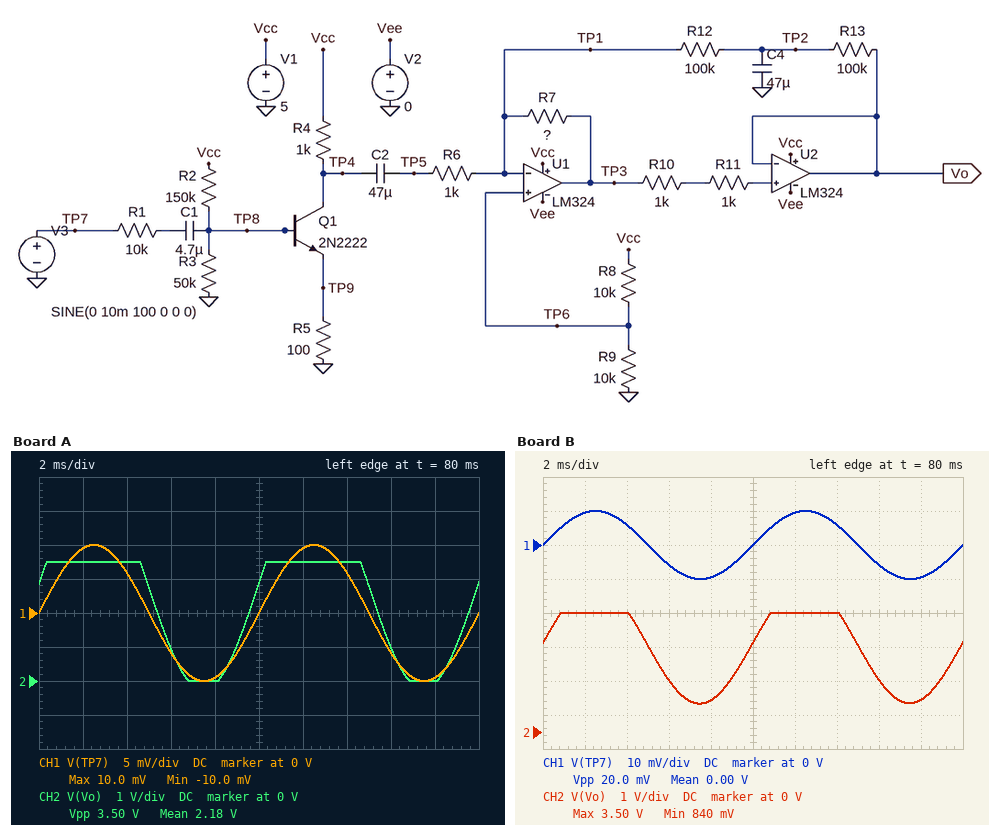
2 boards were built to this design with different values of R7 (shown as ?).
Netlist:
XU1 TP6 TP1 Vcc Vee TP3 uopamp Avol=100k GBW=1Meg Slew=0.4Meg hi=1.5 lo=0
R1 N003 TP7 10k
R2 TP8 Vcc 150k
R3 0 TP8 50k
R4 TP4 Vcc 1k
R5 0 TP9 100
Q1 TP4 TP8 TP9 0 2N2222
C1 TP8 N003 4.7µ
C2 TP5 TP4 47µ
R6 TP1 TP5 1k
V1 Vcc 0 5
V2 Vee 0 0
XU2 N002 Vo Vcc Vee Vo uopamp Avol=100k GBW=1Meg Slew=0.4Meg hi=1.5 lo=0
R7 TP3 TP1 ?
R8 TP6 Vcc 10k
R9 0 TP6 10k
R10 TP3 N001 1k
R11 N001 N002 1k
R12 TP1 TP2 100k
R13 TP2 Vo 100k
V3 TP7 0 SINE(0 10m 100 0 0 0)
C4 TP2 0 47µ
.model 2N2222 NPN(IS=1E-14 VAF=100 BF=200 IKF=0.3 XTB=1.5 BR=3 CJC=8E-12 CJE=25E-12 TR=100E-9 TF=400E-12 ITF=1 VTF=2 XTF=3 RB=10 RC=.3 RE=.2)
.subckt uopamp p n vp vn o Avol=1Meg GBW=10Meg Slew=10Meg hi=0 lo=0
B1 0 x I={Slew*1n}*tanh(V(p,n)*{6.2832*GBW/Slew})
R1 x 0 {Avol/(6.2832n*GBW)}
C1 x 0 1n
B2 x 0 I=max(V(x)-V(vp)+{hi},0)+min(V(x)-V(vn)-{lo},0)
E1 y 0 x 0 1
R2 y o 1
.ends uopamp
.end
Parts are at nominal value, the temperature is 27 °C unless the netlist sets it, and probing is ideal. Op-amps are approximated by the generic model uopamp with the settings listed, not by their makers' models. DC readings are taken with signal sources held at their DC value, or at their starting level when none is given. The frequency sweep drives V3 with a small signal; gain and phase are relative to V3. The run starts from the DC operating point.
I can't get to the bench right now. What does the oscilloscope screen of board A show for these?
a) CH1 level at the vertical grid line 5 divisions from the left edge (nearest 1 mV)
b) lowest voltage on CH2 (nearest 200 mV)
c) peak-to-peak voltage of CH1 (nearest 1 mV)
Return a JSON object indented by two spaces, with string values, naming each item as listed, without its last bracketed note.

{
  "CH1 level at the vertical grid line 5 divisions from the left edge": "0 V",
  "lowest voltage on CH2": "0 V",
  "peak-to-peak voltage of CH1": "20 mV"
}
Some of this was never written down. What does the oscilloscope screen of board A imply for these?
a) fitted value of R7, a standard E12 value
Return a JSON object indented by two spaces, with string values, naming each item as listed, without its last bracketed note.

{
  "fitted value of R7, a standard E12 value": "120 kΩ"
}
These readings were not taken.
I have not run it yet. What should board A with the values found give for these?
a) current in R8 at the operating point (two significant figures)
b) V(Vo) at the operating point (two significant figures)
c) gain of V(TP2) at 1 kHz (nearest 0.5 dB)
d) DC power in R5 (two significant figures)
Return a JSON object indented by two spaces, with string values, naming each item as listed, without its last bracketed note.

{
  "current in R8 at the operating point": "250 µA",
  "V(Vo) at the operating point": "2.5 V",
  "gain of V(TP2) at 1 kHz": "-39.5 dB",
  "DC power in R5": "410 µW"
}
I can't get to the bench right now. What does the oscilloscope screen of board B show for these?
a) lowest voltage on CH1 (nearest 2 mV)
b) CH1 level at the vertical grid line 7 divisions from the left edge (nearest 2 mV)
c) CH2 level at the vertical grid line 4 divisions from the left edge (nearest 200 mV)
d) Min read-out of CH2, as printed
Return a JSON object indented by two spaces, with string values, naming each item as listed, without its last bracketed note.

{
  "lowest voltage on CH1": "-10 mV",
  "CH1 level at the vertical grid line 7 divisions from the left edge": "6 mV",
  "CH2 level at the vertical grid line 4 divisions from the left edge": "1.0 V",
  "Min read-out of CH2, as printed": "840 mV"
}
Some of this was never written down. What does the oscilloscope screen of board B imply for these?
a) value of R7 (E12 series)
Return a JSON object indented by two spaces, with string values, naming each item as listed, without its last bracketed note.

{
  "value of R7": "68 kΩ"
}
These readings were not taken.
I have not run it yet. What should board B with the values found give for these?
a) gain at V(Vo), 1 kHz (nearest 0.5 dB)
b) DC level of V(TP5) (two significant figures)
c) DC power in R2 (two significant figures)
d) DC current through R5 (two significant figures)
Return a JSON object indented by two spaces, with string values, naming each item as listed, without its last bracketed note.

{
  "gain at V(Vo), 1 kHz": "45.0 dB",
  "DC level of V(TP5)": "2.5 V",
  "DC power in R2": "110 µW",
  "DC current through R5": "2.0 mA"
}
